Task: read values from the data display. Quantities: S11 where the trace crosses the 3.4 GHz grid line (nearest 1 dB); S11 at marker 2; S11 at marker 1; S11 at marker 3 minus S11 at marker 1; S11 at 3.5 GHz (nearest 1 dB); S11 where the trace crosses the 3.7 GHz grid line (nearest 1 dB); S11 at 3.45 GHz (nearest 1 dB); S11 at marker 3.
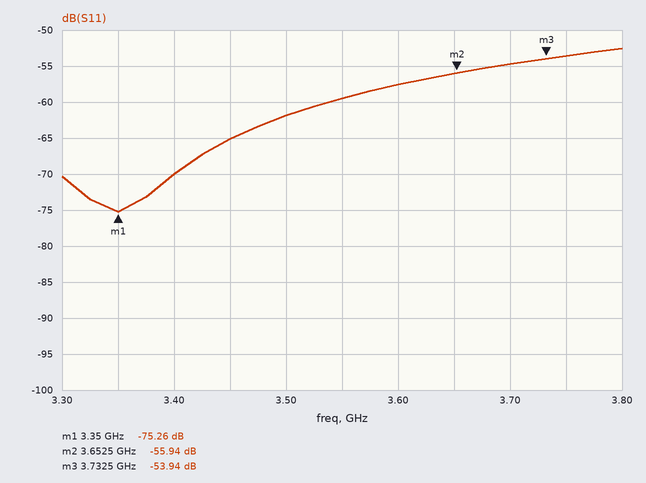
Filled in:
-70 dB
-55.94 dB
-75.26 dB
21.32 dB
-62 dB
-55 dB
-65 dB
-53.94 dB
